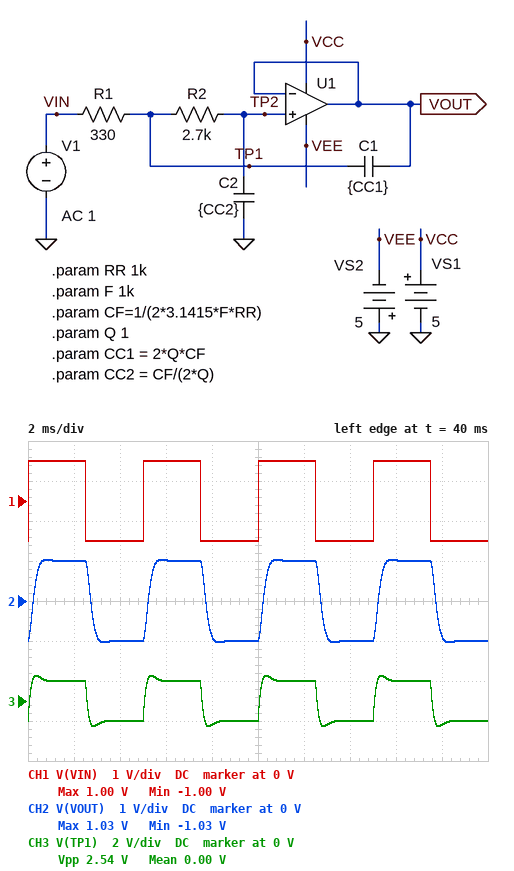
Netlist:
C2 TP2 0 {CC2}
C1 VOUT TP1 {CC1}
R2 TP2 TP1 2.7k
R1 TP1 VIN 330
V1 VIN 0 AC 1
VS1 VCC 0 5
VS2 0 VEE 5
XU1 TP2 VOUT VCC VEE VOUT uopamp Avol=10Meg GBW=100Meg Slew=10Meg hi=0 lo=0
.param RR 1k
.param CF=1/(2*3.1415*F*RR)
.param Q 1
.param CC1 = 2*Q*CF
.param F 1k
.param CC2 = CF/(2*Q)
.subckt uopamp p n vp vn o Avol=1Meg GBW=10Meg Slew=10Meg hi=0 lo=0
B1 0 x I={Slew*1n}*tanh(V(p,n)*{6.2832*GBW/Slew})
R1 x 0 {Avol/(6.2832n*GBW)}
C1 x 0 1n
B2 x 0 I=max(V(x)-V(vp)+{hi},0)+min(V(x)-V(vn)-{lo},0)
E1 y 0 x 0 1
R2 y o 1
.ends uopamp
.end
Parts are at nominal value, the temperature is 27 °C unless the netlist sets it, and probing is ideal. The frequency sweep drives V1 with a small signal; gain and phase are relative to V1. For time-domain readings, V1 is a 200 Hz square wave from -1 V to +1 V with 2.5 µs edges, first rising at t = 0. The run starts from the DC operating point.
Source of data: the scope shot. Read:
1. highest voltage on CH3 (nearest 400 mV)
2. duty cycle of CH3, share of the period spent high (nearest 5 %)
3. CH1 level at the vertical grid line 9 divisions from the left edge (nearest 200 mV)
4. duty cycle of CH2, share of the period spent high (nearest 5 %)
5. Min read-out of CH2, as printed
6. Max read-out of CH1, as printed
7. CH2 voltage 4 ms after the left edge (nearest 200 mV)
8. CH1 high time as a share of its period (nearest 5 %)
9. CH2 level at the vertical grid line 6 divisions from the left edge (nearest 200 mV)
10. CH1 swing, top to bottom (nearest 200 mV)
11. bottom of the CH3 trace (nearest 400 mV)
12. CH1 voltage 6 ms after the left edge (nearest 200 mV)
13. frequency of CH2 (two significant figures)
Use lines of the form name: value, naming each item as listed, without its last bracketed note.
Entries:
highest voltage on CH3: 1.2 V
duty cycle of CH3, share of the period spent high: 50 %
CH1 level at the vertical grid line 9 divisions from the left edge: -1.0 V
duty cycle of CH2, share of the period spent high: 50 %
Min read-out of CH2, as printed: -1.03 V
Max read-out of CH1, as printed: 1.00 V
CH2 voltage 4 ms after the left edge: -1.0 V
CH1 high time as a share of its period: 50 %
CH2 level at the vertical grid line 6 divisions from the left edge: 1.0 V
CH1 swing, top to bottom: 2.0 V
bottom of the CH3 trace: -1.2 V
CH1 voltage 6 ms after the left edge: 1.0 V
frequency of CH2: 200 Hz
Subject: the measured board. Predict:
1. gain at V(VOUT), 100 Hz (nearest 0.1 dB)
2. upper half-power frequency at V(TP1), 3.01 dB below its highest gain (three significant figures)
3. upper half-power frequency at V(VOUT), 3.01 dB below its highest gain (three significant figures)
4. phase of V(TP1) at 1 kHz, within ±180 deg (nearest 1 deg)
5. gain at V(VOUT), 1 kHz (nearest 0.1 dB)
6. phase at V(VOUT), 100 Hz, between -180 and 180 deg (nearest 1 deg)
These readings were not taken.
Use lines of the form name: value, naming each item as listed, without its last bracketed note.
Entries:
gain at V(VOUT), 100 Hz: 0 dB
upper half-power frequency at V(TP1), 3.01 dB below its highest gain: 1.75 kHz
upper half-power frequency at V(VOUT), 3.01 dB below its highest gain: 919 Hz
phase of V(TP1) at 1 kHz, within ±180 deg: -32 deg
gain at V(VOUT), 1 kHz: -3.6 dB
phase at V(VOUT), 100 Hz, between -180 and 180 deg: -9 deg
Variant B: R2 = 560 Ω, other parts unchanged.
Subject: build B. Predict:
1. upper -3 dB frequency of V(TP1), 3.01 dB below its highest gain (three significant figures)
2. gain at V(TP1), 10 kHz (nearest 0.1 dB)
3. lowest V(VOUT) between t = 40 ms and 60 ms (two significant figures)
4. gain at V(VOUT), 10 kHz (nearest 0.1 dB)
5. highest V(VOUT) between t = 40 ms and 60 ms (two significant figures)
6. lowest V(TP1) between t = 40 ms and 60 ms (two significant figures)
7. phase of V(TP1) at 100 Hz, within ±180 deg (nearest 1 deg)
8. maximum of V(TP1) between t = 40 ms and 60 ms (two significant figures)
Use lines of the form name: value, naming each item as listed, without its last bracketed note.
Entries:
upper -3 dB frequency of V(TP1), 3.01 dB below its highest gain: 2.98 kHz
gain at V(TP1), 10 kHz: -15.7 dB
lowest V(VOUT) between t = 40 ms and 60 ms: -1.3 V
gain at V(VOUT), 10 kHz: -25.1 dB
highest V(VOUT) between t = 40 ms and 60 ms: 1.3 V
lowest V(TP1) between t = 40 ms and 60 ms: -1.4 V
phase of V(TP1) at 100 Hz, within ±180 deg: -1 deg
maximum of V(TP1) between t = 40 ms and 60 ms: 1.4 V
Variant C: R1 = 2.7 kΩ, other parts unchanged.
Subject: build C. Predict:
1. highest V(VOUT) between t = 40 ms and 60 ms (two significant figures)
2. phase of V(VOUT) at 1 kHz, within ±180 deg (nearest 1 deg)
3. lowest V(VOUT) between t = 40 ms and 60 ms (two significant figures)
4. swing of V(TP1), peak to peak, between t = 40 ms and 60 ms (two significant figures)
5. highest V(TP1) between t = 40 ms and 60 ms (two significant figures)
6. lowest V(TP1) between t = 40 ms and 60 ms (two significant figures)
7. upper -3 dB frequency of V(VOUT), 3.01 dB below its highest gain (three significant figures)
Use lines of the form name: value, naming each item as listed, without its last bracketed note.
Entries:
highest V(VOUT) between t = 40 ms and 60 ms: 1.3 V
phase of V(VOUT) at 1 kHz, within ±180 deg: -157 deg
lowest V(VOUT) between t = 40 ms and 60 ms: -1.3 V
swing of V(TP1), peak to peak, between t = 40 ms and 60 ms: 2.8 V
highest V(TP1) between t = 40 ms and 60 ms: 1.4 V
lowest V(TP1) between t = 40 ms and 60 ms: -1.4 V
upper -3 dB frequency of V(VOUT), 3.01 dB below its highest gain: 433 Hz
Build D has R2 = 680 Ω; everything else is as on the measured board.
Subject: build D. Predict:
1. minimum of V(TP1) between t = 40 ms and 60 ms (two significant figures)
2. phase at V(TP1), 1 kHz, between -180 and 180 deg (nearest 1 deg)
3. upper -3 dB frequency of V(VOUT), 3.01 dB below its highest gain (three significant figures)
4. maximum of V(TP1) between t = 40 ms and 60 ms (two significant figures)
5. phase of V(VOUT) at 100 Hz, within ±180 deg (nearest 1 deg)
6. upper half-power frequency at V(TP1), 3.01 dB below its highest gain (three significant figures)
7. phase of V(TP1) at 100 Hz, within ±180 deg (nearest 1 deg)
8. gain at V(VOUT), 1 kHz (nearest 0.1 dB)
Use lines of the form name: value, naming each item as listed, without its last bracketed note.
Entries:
minimum of V(TP1) between t = 40 ms and 60 ms: -1.4 V
phase at V(TP1), 1 kHz, between -180 and 180 deg: -14 deg
upper -3 dB frequency of V(VOUT), 3.01 dB below its highest gain: 2.44 kHz
maximum of V(TP1) between t = 40 ms and 60 ms: 1.4 V
phase of V(VOUT) at 100 Hz, within ±180 deg: -3 deg
upper half-power frequency at V(TP1), 3.01 dB below its highest gain: 2.75 kHz
phase of V(TP1) at 100 Hz, within ±180 deg: -1 deg
gain at V(VOUT), 1 kHz: 0.7 dB
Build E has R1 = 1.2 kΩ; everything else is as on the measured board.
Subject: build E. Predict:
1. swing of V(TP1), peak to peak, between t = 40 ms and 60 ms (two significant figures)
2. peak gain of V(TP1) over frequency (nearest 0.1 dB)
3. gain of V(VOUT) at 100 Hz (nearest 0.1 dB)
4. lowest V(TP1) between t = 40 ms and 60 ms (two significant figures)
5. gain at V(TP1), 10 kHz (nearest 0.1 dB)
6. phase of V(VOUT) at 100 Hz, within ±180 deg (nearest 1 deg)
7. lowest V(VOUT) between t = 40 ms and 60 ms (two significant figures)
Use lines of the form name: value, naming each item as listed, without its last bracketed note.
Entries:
swing of V(TP1), peak to peak, between t = 40 ms and 60 ms: 2.8 V
peak gain of V(TP1) over frequency: 1.9 dB
gain of V(VOUT) at 100 Hz: 0.1 dB
lowest V(TP1) between t = 40 ms and 60 ms: -1.4 V
gain at V(TP1), 10 kHz: -27.6 dB
phase of V(VOUT) at 100 Hz, within ±180 deg: -11 deg
lowest V(VOUT) between t = 40 ms and 60 ms: -1.3 V
